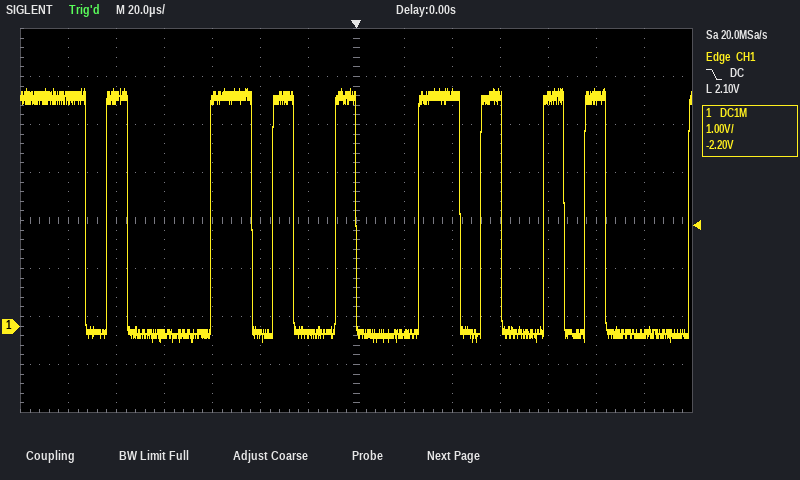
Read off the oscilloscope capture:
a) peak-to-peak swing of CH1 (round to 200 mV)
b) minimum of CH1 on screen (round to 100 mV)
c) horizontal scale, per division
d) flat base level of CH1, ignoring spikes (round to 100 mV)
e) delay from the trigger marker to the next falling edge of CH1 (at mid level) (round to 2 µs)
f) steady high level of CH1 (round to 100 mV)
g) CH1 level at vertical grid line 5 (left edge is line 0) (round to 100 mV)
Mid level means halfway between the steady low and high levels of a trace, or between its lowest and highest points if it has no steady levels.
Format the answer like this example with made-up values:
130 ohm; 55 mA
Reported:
5.2 V; -300 mV; 20 µs; -200 mV; 44 µs; 4.8 V; -200 mV
